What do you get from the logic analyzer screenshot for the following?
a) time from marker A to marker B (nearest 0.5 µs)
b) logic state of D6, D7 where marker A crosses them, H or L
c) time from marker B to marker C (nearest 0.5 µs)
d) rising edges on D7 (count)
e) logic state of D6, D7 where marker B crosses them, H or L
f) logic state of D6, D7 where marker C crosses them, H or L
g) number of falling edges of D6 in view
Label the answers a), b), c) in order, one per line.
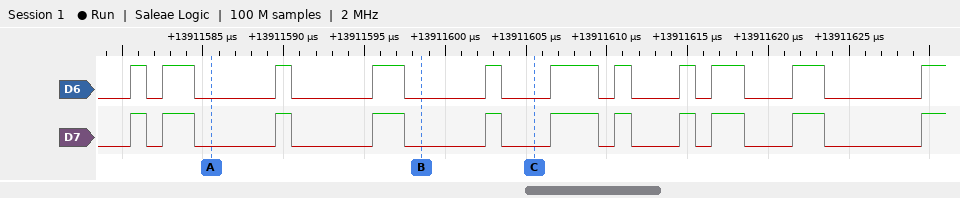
a) 13 µs
b) D6=L, D7=L
c) 7 µs
d) 11
e) D6=L, D7=L
f) D6=L, D7=L
g) 10
